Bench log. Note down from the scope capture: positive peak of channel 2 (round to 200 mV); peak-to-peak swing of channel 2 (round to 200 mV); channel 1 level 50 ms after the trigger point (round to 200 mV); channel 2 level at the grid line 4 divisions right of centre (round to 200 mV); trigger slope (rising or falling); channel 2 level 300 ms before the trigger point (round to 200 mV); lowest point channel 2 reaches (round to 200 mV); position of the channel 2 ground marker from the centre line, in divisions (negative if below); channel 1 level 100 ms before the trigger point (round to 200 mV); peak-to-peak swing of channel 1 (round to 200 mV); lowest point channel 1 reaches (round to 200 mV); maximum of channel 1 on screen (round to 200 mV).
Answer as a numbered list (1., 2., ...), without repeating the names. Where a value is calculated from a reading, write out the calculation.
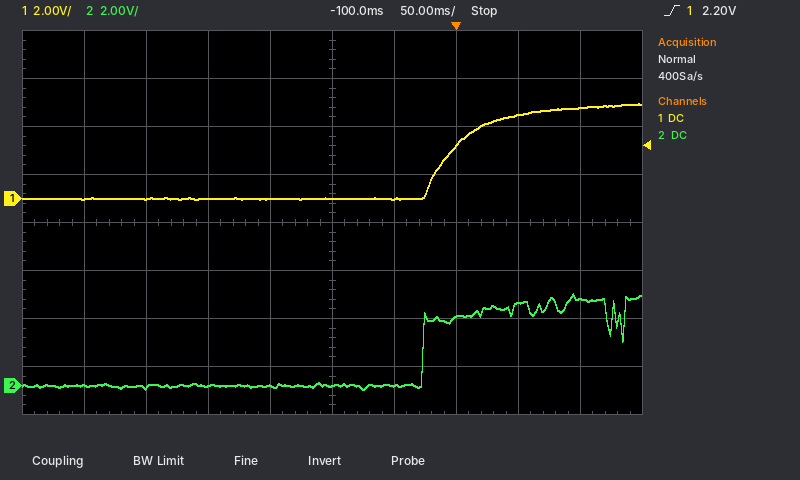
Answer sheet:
1. 3.8 V
2. 3.8 V − (-200 mV) = 4.0 V
3. 3.4 V
4. 3.6 V
5. rising
6. 0.0 V
7. -200 mV
8. -3.4 div
9. 0.0 V
10. 4.0 V − (0.0 V) = 4.0 V
11. 0.0 V
12. 4.0 V
